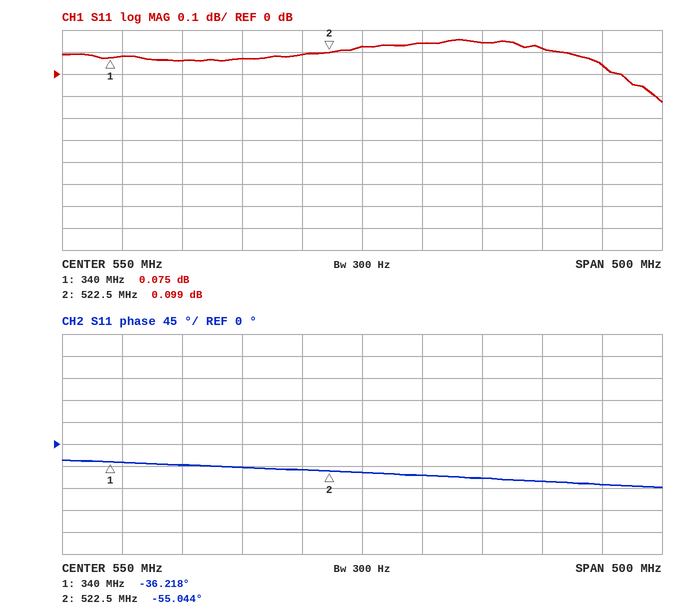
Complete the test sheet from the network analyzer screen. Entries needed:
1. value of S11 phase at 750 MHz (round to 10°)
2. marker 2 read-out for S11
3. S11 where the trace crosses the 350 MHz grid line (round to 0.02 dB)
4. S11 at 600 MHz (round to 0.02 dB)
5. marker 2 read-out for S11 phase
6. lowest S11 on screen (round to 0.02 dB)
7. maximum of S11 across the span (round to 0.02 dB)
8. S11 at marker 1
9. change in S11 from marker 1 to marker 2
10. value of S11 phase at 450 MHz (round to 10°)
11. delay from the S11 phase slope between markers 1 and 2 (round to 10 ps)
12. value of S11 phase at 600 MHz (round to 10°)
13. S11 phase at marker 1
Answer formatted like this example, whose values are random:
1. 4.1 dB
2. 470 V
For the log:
1. -80°
2. 0.099 dB
3. 0.08 dB
4. 0.14 dB
5. -55.044°
6. -0.12 dB
7. 0.16 dB
8. 0.075 dB
9. 0.024 dB
10. -50°
11. 290 ps
12. -60°
13. -36.218°
